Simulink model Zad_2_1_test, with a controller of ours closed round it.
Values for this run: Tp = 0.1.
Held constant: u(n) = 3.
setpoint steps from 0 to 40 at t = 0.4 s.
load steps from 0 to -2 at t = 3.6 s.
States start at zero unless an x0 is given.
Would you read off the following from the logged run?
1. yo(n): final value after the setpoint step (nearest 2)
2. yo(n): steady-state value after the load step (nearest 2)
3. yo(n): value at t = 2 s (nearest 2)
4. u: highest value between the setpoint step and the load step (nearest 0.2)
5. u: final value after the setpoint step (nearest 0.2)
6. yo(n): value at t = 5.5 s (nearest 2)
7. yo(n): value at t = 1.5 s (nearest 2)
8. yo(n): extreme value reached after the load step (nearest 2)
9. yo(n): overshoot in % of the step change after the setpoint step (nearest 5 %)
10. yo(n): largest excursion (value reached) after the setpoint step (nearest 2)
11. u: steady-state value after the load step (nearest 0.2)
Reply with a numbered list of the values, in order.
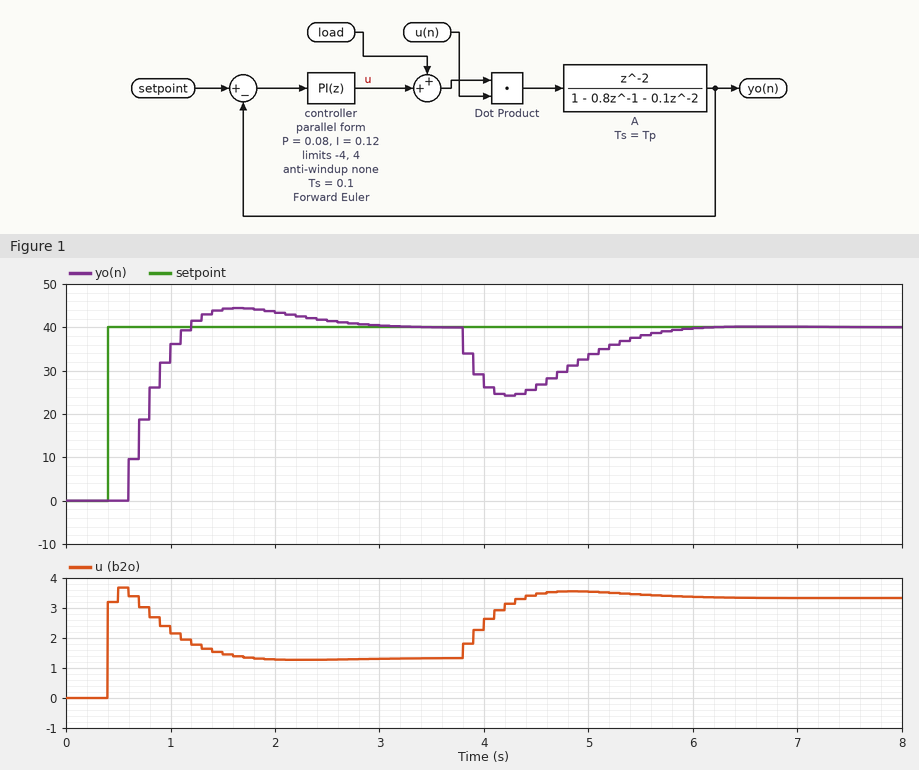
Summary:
1. 40
2. 40
3. 44
4. 3.6
5. 1.4
6. 38
7. 44
8. 24
9. 10 %
10. 44
11. 3.4
